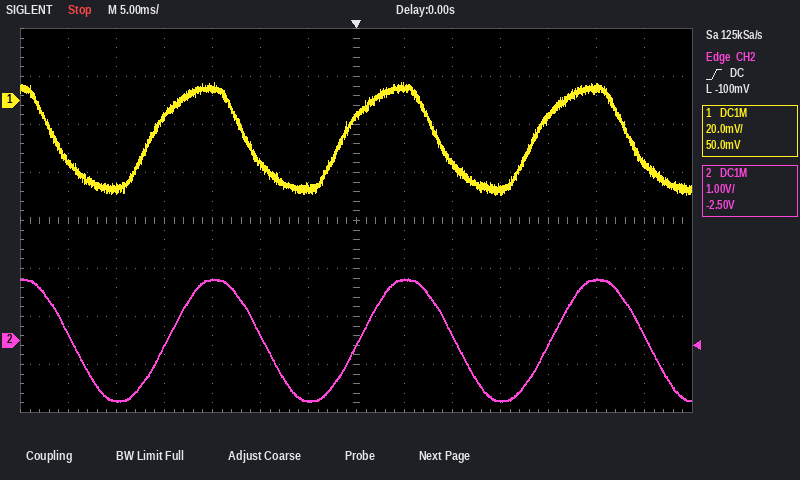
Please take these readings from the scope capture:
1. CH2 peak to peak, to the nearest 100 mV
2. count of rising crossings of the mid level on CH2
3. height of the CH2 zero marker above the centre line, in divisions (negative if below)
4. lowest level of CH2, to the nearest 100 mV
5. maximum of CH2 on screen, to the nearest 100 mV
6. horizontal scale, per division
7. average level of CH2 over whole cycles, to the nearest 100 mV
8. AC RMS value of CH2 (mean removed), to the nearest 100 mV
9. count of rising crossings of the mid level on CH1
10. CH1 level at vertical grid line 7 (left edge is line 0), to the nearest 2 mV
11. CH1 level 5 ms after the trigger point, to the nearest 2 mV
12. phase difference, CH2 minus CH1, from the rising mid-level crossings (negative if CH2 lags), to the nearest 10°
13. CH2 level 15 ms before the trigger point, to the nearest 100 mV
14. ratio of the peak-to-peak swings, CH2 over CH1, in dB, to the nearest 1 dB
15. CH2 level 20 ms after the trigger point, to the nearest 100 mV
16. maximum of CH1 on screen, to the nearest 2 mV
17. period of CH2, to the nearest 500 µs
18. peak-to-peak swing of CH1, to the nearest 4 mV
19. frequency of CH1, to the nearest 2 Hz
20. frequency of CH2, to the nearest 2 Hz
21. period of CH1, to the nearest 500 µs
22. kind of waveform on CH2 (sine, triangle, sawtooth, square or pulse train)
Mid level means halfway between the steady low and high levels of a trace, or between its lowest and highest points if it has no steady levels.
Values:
2.6 V
3
-2.5 div
-1.3 V
1.3 V
5 ms
0.0 V
900 mV
3
-6 mV
6 mV
-30°
1.3 V
35 dB
-100 mV
8 mV
20.0 ms
48 mV
50 Hz
50 Hz
20.0 ms
sine
